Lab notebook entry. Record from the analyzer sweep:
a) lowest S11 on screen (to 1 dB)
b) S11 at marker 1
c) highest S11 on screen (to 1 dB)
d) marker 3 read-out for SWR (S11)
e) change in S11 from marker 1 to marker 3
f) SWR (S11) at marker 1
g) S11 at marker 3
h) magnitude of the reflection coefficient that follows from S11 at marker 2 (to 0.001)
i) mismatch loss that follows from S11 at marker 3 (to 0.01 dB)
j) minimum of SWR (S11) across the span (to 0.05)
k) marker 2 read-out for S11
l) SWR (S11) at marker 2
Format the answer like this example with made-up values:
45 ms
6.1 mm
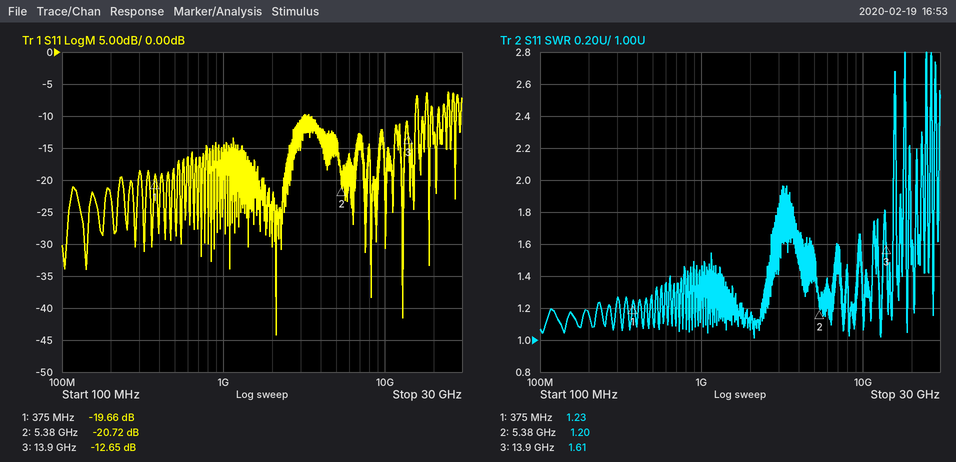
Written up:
-44 dB
-19.66 dB
-6 dB
1.61
7.01 dB
1.23
-12.65 dB
0.092
0.24 dB
1.00
-20.72 dB
1.20
